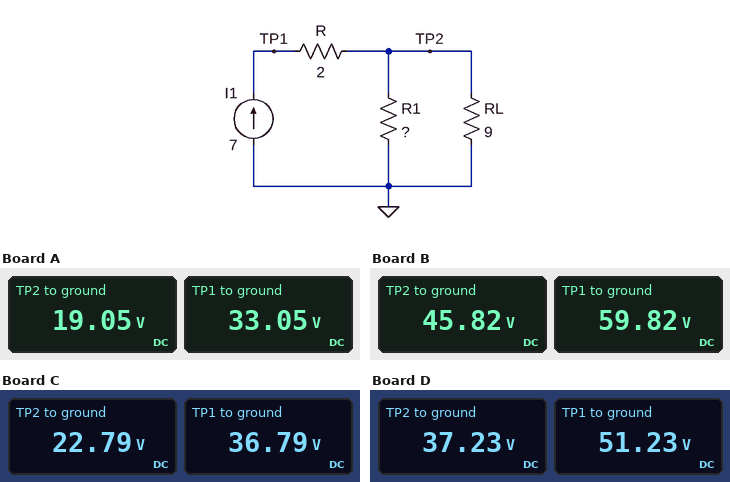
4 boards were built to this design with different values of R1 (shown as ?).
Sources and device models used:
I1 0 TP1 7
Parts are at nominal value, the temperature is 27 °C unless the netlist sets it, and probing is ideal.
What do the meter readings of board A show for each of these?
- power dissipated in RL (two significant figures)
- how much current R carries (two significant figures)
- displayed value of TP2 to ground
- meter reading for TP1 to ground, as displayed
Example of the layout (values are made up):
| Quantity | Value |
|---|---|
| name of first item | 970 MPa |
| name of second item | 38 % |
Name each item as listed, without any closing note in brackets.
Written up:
| Quantity | Value |
|---|---|
| power dissipated in RL | 40 W |
| how much current R carries | 7.0 A |
| displayed value of TP2 to ground | 19.05 V |
| meter reading for TP1 to ground, as displayed | 33.05 V |
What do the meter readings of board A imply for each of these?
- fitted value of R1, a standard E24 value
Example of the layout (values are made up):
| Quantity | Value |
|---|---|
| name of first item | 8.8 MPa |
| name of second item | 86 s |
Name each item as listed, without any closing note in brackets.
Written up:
| Quantity | Value |
|---|---|
| fitted value of R1, a standard E24 value | 3.9 Ω |
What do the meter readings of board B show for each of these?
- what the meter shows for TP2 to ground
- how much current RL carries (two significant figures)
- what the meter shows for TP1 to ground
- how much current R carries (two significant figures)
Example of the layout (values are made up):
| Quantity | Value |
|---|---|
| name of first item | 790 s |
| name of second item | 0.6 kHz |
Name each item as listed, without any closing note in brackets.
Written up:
| Quantity | Value |
|---|---|
| what the meter shows for TP2 to ground | 45.82 V |
| how much current RL carries | 5.1 A |
| what the meter shows for TP1 to ground | 59.82 V |
| how much current R carries | 7.0 A |
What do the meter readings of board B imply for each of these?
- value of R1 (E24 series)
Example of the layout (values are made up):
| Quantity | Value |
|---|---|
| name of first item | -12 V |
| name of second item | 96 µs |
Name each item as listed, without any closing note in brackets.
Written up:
| Quantity | Value |
|---|---|
| value of R1 | 24 Ω |
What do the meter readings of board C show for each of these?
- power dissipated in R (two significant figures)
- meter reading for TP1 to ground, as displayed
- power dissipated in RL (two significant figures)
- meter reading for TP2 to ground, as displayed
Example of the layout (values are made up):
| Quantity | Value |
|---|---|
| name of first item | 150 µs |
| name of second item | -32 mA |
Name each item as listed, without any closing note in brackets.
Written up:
| Quantity | Value |
|---|---|
| power dissipated in R | 98 W |
| meter reading for TP1 to ground, as displayed | 36.79 V |
| power dissipated in RL | 58 W |
| meter reading for TP2 to ground, as displayed | 22.79 V |
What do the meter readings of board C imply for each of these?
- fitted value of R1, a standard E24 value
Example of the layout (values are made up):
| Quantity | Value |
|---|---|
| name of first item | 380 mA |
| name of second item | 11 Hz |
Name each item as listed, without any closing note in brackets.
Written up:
| Quantity | Value |
|---|---|
| fitted value of R1, a standard E24 value | 5.1 Ω |
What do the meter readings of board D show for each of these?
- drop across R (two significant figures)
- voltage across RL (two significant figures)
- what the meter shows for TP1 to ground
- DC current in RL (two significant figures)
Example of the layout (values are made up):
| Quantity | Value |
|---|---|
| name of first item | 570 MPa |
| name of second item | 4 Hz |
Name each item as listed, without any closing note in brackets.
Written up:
| Quantity | Value |
|---|---|
| drop across R | 14 V |
| voltage across RL | 37 V |
| what the meter shows for TP1 to ground | 51.23 V |
| DC current in RL | 4.1 A |
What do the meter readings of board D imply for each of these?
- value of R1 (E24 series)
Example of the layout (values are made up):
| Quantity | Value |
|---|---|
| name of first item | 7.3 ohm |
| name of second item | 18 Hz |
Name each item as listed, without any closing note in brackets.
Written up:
| Quantity | Value |
|---|---|
| value of R1 | 13 Ω |
